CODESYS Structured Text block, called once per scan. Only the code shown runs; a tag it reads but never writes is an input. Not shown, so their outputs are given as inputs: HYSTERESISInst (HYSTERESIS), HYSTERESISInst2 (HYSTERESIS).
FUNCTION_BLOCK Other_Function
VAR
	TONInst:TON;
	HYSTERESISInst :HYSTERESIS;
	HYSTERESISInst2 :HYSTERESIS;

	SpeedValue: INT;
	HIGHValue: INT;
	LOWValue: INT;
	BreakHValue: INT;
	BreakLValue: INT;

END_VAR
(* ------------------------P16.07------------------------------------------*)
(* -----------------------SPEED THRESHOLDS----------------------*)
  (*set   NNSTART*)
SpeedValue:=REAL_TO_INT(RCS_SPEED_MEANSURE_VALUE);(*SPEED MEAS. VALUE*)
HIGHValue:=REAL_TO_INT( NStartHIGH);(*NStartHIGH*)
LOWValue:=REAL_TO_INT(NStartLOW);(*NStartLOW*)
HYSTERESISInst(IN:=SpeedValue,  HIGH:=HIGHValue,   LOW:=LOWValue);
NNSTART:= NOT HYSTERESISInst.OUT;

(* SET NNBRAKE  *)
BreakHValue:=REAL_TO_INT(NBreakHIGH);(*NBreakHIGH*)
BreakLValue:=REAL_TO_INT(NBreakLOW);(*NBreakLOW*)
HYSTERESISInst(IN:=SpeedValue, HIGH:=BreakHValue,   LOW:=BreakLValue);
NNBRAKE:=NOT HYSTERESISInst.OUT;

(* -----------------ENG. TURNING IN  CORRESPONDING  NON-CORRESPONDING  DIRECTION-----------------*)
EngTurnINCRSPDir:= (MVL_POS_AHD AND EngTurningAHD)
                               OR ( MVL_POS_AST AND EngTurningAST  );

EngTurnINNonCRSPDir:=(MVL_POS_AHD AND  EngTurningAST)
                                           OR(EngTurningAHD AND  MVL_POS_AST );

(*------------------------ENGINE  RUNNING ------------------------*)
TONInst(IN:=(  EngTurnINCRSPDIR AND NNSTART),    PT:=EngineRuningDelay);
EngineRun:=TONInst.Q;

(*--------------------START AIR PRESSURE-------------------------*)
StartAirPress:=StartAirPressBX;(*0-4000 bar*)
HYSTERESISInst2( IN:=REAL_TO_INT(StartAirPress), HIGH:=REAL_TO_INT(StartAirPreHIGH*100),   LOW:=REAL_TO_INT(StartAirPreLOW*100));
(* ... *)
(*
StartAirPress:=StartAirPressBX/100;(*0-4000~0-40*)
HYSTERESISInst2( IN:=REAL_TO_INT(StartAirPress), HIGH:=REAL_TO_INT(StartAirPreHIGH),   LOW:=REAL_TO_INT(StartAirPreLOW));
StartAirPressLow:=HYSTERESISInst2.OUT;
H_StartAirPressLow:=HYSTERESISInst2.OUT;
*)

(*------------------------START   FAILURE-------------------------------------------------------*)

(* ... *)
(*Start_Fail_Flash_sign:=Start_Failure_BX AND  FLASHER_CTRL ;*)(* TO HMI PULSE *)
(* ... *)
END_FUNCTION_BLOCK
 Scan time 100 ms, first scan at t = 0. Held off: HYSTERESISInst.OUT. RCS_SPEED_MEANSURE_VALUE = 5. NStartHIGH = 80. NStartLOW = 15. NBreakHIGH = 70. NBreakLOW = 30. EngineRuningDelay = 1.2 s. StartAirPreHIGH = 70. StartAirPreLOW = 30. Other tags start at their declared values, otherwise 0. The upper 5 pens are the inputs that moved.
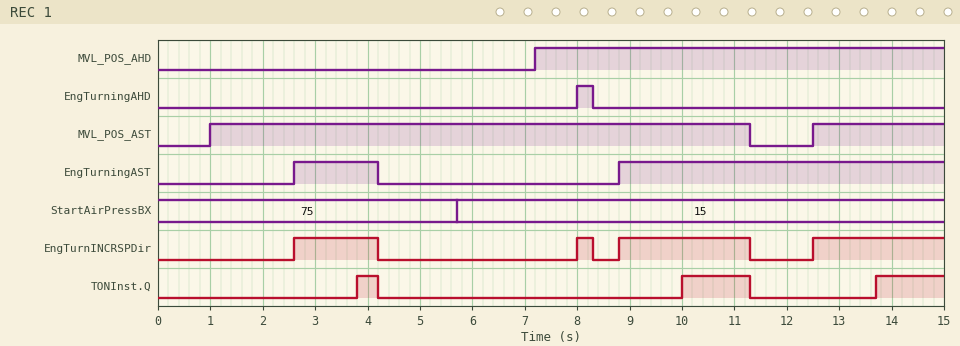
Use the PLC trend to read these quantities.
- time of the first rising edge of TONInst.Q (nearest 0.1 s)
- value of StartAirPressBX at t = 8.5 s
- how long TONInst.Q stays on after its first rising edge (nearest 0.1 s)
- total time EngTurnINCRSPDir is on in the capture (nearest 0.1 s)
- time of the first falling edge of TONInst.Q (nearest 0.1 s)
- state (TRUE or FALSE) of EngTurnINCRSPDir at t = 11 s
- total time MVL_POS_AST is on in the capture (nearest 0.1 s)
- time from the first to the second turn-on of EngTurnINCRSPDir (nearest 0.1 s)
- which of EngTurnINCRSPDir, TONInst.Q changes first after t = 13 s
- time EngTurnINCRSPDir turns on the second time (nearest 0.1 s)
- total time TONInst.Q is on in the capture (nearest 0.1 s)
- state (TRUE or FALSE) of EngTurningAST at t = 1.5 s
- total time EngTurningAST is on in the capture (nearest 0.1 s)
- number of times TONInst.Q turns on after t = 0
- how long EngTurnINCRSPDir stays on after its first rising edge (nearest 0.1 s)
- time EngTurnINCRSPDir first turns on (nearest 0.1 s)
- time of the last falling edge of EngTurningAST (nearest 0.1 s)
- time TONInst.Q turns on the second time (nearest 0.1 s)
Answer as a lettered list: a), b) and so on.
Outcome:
a) 3.8 s
b) 15
c) 0.4 s
d) 6.9 s
e) 4.2 s
f) TRUE
g) 12.8 s
h) 5.4 s
i) TONInst.Q
j) 8.0 s
k) 3.0 s
l) FALSE
m) 7.8 s
n) 3
o) 1.6 s
p) 2.6 s
q) 4.2 s
r) 10.0 s
